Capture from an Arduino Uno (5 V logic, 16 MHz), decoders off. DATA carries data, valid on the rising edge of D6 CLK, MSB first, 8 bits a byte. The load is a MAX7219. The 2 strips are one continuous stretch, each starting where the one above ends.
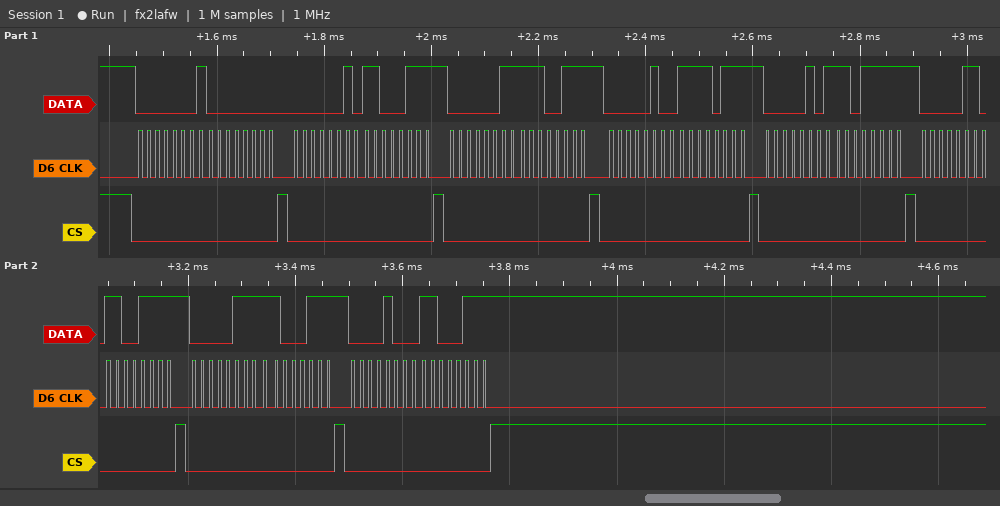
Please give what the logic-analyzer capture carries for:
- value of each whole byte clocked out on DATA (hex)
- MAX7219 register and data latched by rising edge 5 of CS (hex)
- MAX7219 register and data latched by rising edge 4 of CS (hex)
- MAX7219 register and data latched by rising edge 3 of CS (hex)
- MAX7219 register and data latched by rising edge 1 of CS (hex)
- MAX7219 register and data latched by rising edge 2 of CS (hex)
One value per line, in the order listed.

0x01 0x00 0x02 0xC7 0x03 0xE7 0x04 0xF7 0x05 0xDF 0x06 0xCF 0x07 0xC7 0x08 0xC7
register 0x5, data 0xDF
register 0x4, data 0xF7
register 0x3, data 0xE7
register 0x1, data 0x00
register 0x2, data 0xC7
